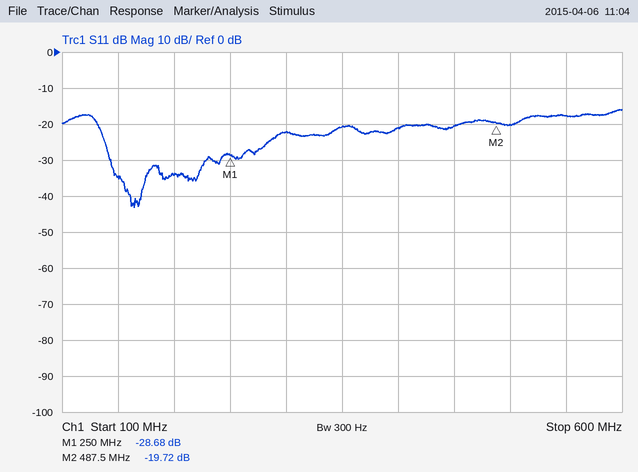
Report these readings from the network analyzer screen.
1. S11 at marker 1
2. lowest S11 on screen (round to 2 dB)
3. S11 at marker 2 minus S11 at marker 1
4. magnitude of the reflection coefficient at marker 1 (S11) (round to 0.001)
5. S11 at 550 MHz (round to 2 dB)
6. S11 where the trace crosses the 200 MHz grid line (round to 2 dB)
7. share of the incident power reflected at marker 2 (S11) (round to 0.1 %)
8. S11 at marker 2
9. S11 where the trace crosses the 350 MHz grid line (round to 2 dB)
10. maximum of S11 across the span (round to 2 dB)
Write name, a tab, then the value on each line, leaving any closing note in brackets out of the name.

S11 at marker 1	-28.68 dB
lowest S11 on screen	-44 dB
S11 at marker 2 minus S11 at marker 1	8.96 dB
magnitude of the reflection coefficient at marker 1 (S11)	0.037
S11 at 550 MHz	-18 dB
S11 where the trace crosses the 200 MHz grid line	-34 dB
share of the incident power reflected at marker 2 (S11)	1.1 %
S11 at marker 2	-19.72 dB
S11 where the trace crosses the 350 MHz grid line	-20 dB
maximum of S11 across the span	-16 dB
